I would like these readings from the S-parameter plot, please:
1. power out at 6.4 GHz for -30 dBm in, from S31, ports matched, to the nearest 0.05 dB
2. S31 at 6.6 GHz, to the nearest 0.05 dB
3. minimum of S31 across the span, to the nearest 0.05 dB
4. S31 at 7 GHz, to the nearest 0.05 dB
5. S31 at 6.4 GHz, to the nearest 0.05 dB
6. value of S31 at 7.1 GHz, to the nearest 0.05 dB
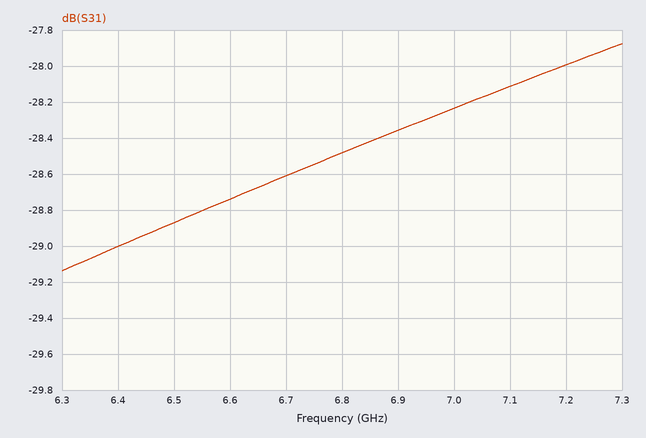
-59.00 dBm
-28.75 dB
-29.15 dB
-28.25 dB
-29.00 dB
-28.10 dB
